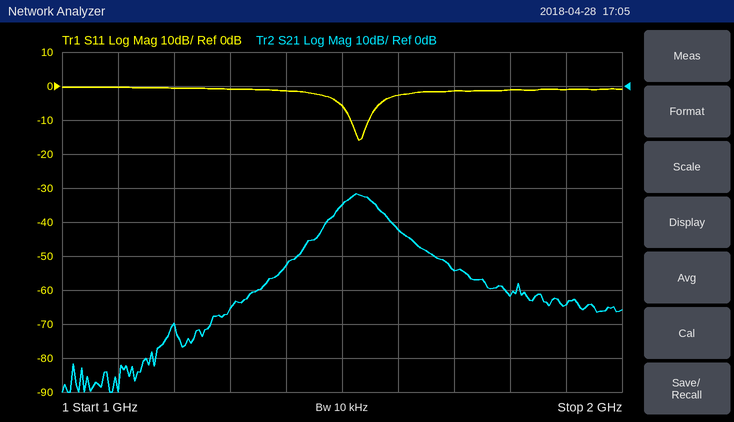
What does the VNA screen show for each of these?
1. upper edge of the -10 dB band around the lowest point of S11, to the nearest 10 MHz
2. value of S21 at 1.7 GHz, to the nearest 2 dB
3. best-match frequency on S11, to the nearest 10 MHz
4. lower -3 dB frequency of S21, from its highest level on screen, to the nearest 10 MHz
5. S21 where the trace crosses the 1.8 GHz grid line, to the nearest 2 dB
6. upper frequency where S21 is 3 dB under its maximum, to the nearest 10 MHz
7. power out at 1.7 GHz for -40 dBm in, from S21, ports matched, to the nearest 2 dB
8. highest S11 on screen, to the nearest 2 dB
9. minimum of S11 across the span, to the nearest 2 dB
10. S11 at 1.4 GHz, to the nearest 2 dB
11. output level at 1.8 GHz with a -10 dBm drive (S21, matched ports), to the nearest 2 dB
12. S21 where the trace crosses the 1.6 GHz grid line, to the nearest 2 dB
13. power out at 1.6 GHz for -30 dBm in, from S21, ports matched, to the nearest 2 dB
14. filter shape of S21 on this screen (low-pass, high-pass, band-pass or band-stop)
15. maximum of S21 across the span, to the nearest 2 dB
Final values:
1.55 GHz
-54 dB
1.53 GHz
1.50 GHz
-62 dB
1.56 GHz
-94 dBm
0 dB
-16 dB
-2 dB
-72 dBm
-42 dB
-72 dBm
band-pass
-32 dB
